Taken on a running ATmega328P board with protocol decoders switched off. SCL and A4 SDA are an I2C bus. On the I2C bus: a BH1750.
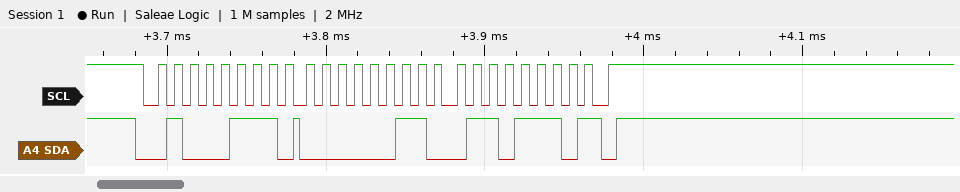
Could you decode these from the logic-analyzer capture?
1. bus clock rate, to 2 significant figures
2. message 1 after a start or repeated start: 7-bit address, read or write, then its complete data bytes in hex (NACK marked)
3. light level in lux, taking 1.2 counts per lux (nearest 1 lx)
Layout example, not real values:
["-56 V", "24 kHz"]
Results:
["100 kHz", "0x23 read: 03 6E NACK", "732 lx"]
